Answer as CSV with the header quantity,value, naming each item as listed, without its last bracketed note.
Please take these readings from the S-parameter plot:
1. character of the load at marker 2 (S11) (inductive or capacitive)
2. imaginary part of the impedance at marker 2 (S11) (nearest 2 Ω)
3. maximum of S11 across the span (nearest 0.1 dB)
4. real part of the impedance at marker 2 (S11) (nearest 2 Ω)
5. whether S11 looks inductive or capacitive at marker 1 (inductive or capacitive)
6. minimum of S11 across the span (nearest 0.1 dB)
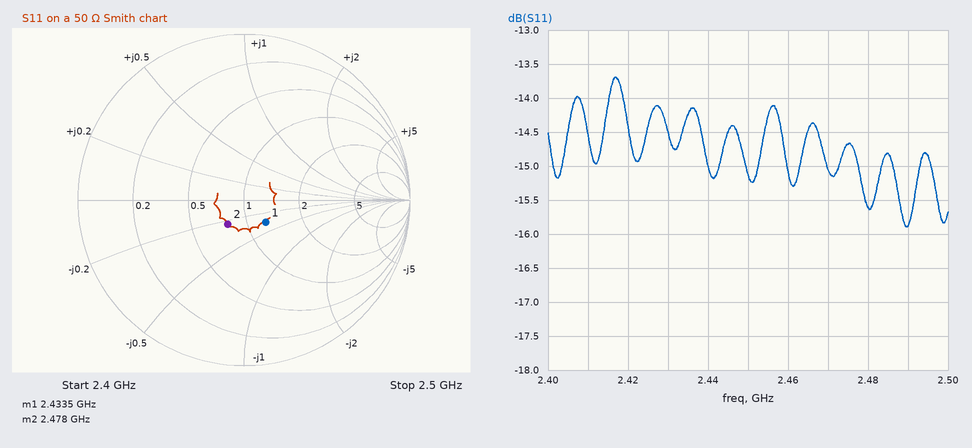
quantity,value
character of the load at marker 2 (S11),capacitive
imaginary part of the impedance at marker 2 (S11),-12 Ω
maximum of S11 across the span,-13.7 dB
real part of the impedance at marker 2 (S11),40 Ω
whether S11 looks inductive or capacitive at marker 1,capacitive
minimum of S11 across the span,-15.9 dB
